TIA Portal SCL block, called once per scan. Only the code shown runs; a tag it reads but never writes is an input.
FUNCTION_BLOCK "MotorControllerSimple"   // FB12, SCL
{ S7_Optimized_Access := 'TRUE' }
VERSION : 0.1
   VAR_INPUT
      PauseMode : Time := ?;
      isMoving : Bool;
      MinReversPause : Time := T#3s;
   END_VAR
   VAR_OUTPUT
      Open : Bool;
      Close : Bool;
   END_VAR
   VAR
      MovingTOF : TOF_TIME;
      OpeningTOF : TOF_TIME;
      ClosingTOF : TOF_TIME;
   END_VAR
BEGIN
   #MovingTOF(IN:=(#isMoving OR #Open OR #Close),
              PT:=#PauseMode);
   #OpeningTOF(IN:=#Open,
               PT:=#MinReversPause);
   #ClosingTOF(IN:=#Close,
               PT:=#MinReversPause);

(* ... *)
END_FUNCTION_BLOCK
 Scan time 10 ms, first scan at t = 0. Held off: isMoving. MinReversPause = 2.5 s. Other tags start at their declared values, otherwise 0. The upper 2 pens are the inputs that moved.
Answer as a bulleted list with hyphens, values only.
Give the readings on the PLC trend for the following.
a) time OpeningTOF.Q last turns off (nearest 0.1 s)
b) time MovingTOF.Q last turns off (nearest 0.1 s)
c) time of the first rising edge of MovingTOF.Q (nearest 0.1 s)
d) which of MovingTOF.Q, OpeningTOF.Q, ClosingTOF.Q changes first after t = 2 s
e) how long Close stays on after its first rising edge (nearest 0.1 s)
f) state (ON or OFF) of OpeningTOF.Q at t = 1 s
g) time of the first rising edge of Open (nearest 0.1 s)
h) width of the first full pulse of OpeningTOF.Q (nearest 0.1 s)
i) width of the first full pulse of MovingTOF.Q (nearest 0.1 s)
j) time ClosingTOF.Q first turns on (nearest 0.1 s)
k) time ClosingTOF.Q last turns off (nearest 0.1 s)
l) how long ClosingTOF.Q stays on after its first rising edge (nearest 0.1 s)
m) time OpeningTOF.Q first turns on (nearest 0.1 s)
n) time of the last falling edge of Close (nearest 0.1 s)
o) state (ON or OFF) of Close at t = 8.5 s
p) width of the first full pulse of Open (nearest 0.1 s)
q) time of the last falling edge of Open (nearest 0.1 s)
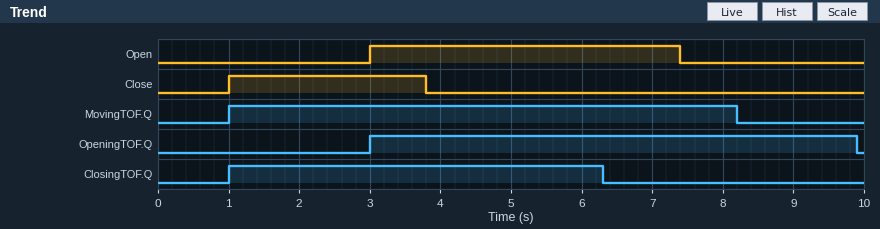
- 9.9 s
- 8.2 s
- 1.0 s
- OpeningTOF.Q
- 2.8 s
- OFF
- 3.0 s
- 6.9 s
- 7.2 s
- 1.0 s
- 6.3 s
- 5.3 s
- 3.0 s
- 3.8 s
- OFF
- 4.4 s
- 7.4 s
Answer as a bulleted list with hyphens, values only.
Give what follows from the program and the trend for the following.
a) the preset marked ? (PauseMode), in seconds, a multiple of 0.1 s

- 0.8 s
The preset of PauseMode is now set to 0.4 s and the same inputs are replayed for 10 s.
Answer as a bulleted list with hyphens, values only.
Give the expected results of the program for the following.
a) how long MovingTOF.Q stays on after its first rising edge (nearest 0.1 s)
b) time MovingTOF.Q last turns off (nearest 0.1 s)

- 6.8 s
- 7.8 s
